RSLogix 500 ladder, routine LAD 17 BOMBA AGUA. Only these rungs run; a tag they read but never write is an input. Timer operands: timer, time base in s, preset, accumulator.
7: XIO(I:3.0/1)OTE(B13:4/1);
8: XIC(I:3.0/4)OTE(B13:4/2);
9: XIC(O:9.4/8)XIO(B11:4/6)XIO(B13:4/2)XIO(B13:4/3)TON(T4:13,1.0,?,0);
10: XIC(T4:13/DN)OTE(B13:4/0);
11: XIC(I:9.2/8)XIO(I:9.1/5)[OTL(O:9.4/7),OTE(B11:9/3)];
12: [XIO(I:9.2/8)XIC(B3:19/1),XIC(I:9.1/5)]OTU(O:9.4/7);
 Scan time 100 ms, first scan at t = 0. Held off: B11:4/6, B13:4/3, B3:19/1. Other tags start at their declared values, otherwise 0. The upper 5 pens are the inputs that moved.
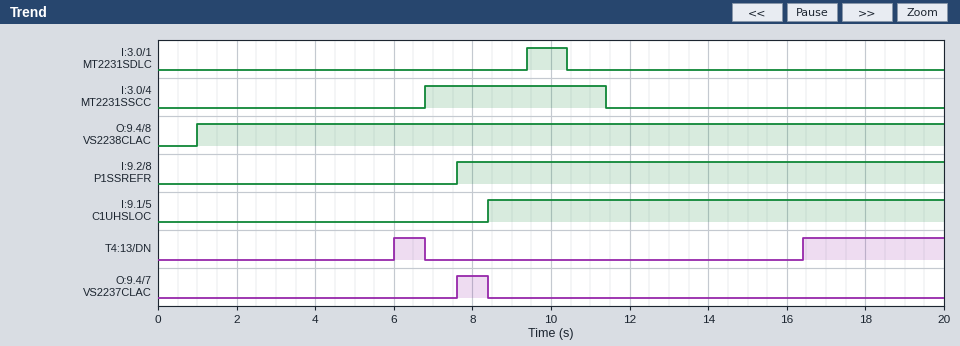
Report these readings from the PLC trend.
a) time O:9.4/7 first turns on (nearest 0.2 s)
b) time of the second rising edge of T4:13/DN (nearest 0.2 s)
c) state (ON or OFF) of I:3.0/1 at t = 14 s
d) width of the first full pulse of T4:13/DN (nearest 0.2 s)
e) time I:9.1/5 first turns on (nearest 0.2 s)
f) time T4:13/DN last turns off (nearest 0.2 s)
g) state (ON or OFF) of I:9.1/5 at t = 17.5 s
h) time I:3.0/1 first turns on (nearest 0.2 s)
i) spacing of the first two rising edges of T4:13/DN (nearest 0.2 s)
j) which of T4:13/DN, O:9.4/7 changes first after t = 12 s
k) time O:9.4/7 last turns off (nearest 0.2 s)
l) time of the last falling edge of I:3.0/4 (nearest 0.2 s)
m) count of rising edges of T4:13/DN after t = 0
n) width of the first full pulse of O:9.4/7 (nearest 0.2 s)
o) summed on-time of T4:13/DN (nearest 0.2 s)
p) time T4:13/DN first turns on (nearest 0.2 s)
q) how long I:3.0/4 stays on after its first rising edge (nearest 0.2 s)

7.6 s
16.4 s
OFF
0.8 s
8.4 s
6.8 s
ON
9.4 s
10.4 s
T4:13/DN
8.4 s
11.4 s
2
0.8 s
4.4 s
6.0 s
4.6 s
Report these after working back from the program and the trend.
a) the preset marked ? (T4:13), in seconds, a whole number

5 s
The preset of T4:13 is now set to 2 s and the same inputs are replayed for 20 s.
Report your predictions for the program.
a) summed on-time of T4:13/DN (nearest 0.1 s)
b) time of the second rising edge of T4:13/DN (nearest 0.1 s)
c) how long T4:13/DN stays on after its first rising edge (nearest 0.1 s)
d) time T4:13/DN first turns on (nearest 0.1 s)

10.4 s
13.4 s
3.8 s
3.0 s
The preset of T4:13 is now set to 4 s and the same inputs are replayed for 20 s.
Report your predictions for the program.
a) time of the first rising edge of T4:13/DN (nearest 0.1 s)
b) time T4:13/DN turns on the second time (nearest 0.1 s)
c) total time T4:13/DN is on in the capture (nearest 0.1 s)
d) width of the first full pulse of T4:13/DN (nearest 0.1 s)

5.0 s
15.4 s
6.4 s
1.8 s
